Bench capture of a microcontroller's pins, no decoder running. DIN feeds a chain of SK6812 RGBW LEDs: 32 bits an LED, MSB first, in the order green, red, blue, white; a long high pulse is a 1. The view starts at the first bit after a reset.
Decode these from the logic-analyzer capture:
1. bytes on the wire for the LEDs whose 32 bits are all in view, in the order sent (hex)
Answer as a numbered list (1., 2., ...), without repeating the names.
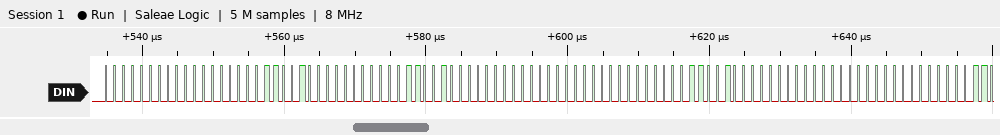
1. 00 00 32 00 32 00 00 00 32 00 00 00
